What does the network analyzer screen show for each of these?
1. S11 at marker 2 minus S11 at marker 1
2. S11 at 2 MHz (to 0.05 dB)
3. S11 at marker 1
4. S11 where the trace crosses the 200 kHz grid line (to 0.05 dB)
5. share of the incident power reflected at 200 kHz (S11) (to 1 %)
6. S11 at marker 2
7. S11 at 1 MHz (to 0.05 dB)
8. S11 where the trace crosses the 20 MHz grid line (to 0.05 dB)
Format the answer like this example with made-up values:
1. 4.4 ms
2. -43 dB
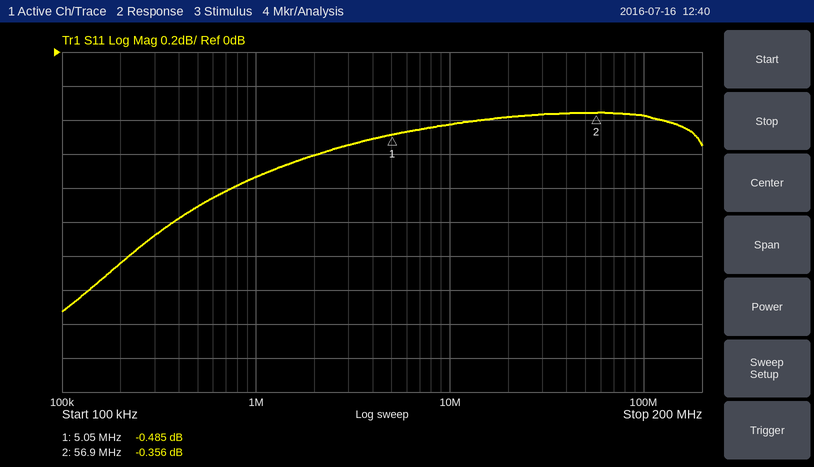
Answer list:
1. 0.129 dB
2. -0.60 dB
3. -0.485 dB
4. -1.25 dB
5. 75 %
6. -0.356 dB
7. -0.75 dB
8. -0.40 dB
